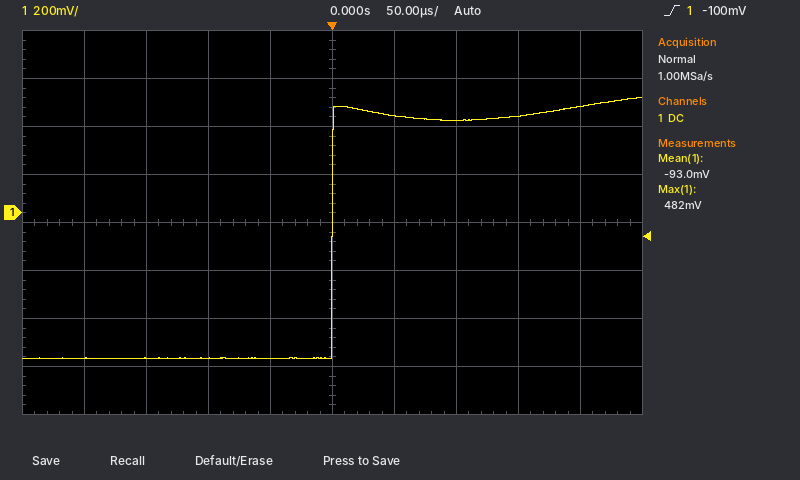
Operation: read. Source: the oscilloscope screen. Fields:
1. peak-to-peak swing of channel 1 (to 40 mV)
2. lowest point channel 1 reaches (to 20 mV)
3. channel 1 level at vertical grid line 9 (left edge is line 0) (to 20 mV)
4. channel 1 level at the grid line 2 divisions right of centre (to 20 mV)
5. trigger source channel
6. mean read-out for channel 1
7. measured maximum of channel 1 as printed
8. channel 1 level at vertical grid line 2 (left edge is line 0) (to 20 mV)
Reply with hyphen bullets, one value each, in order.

- 1.08 V
- -600 mV
- 440 mV
- 380 mV
- channel 1
- -93.0 mV
- 482 mV
- -600 mV
